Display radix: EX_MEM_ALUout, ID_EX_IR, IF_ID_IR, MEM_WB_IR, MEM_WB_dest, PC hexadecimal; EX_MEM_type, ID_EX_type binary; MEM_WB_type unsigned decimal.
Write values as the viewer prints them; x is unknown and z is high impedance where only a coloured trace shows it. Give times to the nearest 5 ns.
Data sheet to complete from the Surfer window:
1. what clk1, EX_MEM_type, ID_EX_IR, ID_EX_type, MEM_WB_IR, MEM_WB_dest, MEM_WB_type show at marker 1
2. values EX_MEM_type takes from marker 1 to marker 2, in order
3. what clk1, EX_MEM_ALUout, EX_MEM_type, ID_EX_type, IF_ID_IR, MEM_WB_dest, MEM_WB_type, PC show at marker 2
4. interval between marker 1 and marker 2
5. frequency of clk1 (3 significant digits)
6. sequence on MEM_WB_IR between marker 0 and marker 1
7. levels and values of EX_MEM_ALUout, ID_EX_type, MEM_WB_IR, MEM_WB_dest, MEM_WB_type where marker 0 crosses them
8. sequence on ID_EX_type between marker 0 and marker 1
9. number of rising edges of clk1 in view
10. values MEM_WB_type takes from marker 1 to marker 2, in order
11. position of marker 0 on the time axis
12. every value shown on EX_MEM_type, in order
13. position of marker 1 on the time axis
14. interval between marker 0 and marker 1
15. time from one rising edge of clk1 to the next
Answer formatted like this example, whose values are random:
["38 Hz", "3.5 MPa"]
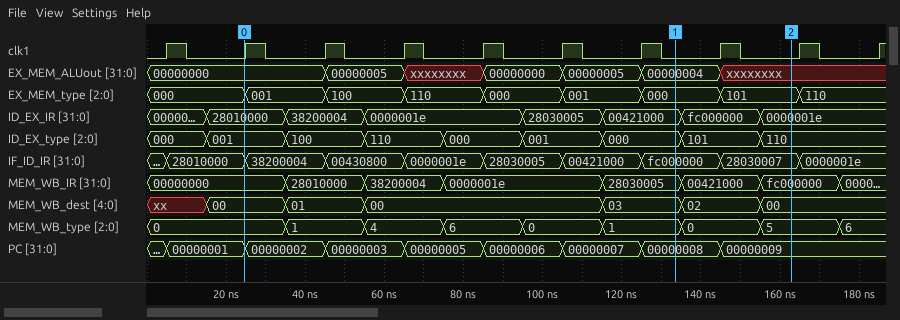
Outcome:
["clk1=0, EX_MEM_type=000, ID_EX_IR=00421000, ID_EX_type=000, MEM_WB_IR=28030005, MEM_WB_dest=03, MEM_WB_type=1", "000, 101", "clk1=0, EX_MEM_ALUout=xxxxxxxx, EX_MEM_type=101, ID_EX_type=110, IF_ID_IR=28030007, MEM_WB_dest=00, MEM_WB_type=5, PC=00000009", "30 ns", "50.0 MHz", "00000000, 28010000, 38200004, 0000001e, 28030005", "EX_MEM_ALUout=00000000, ID_EX_type=001, MEM_WB_IR=00000000, MEM_WB_dest=00, MEM_WB_type=0", "001, 100, 110, 000, 001, 000", "10", "1, 0, 5", "25 ns", "000, 001, 100, 110, 000, 001, 000, 101, 110", "135 ns", "110 ns", "20 ns"]
